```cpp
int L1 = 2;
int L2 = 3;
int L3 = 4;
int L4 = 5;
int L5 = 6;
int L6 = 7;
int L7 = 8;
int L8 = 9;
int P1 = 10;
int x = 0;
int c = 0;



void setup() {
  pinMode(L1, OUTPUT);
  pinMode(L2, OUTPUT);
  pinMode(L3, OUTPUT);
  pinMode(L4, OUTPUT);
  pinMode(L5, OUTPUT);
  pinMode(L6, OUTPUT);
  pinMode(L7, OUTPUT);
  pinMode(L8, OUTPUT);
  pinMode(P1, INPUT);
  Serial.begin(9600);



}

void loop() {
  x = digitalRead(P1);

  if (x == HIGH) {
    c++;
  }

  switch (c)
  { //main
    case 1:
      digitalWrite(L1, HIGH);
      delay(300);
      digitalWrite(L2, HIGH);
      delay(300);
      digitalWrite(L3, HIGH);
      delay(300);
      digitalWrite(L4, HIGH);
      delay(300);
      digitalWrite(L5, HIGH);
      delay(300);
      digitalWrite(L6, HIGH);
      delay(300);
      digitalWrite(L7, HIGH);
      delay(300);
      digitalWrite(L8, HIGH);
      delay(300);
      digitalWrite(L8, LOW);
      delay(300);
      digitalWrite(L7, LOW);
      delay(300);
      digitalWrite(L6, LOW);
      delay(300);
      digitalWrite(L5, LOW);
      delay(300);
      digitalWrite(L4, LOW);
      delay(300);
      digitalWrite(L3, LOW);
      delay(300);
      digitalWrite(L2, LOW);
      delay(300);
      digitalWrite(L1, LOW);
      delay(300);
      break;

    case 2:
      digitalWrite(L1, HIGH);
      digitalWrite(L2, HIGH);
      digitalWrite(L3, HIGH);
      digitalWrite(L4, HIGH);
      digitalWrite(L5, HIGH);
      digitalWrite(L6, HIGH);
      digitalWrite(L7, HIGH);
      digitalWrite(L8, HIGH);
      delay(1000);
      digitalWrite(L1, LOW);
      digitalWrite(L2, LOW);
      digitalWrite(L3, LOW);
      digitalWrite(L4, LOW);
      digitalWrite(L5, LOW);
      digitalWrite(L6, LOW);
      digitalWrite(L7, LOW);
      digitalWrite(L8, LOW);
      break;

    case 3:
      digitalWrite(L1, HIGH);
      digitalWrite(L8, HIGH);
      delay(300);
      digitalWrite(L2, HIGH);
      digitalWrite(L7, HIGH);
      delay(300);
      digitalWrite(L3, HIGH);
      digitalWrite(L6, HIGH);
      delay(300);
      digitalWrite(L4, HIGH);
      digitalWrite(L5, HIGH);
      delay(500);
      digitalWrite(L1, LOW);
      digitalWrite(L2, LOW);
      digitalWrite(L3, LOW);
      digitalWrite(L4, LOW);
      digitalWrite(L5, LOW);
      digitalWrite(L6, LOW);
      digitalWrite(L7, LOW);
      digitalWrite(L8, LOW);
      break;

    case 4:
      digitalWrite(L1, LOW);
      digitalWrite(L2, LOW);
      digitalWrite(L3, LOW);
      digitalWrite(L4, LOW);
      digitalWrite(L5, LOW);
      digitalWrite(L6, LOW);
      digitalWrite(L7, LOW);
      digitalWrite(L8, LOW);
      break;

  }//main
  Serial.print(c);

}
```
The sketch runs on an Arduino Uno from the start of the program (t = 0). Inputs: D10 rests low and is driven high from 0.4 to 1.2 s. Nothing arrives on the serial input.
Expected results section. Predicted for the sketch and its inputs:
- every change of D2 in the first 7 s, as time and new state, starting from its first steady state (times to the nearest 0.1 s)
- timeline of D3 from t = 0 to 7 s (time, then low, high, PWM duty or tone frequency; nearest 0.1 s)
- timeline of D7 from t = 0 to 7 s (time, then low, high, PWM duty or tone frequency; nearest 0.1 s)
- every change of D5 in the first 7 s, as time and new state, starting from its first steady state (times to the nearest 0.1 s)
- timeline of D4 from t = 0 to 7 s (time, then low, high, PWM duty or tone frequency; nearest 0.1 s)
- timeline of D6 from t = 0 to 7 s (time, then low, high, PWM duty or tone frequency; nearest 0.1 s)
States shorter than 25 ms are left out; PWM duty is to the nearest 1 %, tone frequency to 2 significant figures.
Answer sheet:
0 s low; 0.4 s high; 4.9 s low; 5.2 s high
0 s low; 0.7 s high; 4.6 s low; 5.5 s high
0 s low; 1.9 s high; 3.4 s low; 6.7 s high
0 s low; 1.3 s high; 4 s low; 6.1 s high
0 s low; 1 s high; 4.3 s low; 5.8 s high
0 s low; 1.6 s high; 3.7 s low; 6.4 s high
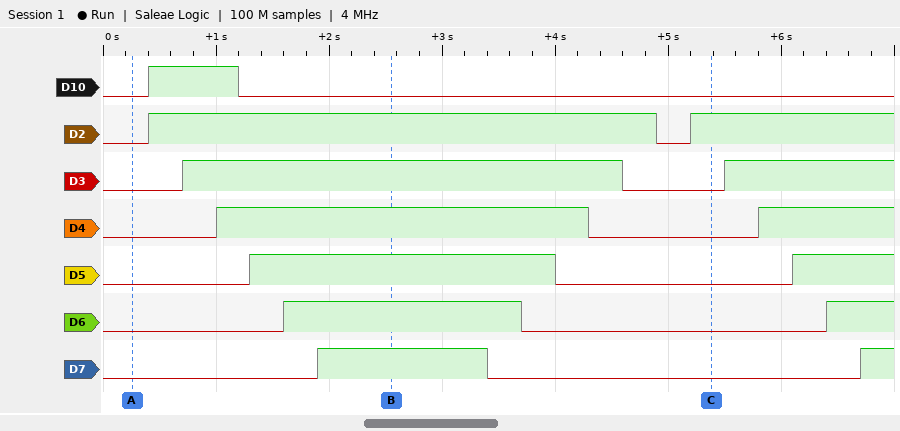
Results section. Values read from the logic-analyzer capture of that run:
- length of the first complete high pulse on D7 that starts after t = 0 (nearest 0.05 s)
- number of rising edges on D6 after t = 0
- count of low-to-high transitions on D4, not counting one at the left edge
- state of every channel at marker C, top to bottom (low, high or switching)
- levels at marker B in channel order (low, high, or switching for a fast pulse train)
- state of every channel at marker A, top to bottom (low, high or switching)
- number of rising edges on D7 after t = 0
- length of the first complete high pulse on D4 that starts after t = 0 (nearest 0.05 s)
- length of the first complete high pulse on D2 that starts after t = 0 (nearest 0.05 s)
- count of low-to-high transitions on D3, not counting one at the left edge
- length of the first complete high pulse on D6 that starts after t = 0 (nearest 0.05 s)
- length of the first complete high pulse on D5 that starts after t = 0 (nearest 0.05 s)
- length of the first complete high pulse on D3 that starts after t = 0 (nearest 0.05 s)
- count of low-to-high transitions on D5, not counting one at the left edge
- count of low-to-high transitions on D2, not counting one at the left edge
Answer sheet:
1.50 s
2
2
D10 low, D2 high, D3 low, D4 low, D5 low, D6 low, D7 low
D10 low, D2 high, D3 high, D4 high, D5 high, D6 high, D7 high
D10 low, D2 low, D3 low, D4 low, D5 low, D6 low, D7 low
2
3.30 s
4.50 s
2
2.10 s
2.70 s
3.90 s
2
2
